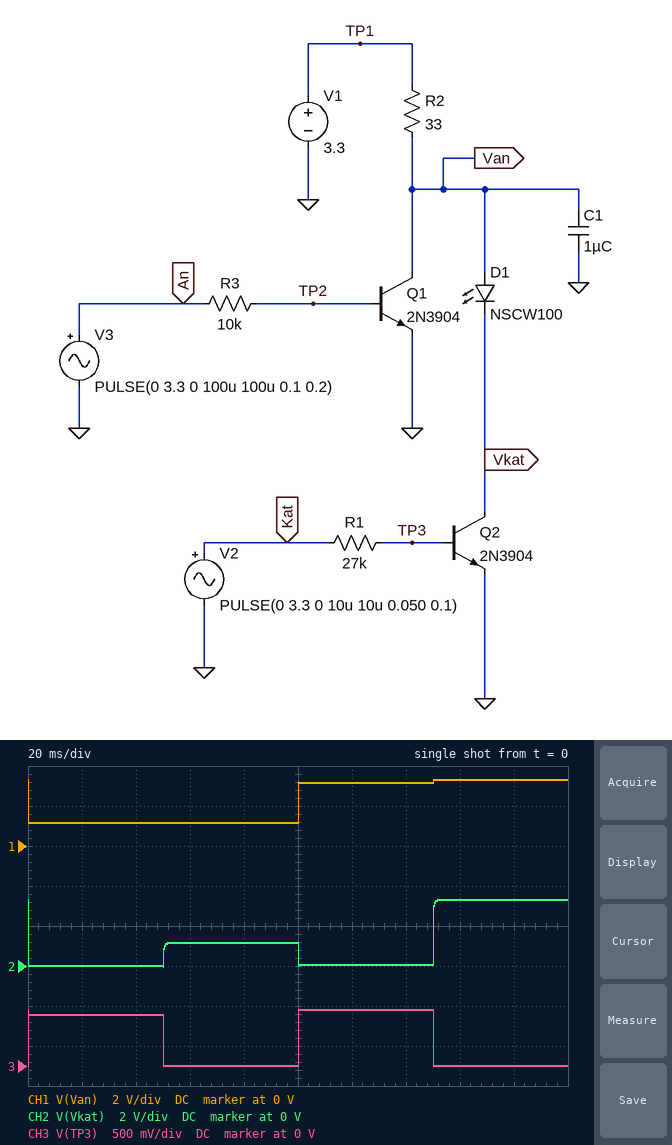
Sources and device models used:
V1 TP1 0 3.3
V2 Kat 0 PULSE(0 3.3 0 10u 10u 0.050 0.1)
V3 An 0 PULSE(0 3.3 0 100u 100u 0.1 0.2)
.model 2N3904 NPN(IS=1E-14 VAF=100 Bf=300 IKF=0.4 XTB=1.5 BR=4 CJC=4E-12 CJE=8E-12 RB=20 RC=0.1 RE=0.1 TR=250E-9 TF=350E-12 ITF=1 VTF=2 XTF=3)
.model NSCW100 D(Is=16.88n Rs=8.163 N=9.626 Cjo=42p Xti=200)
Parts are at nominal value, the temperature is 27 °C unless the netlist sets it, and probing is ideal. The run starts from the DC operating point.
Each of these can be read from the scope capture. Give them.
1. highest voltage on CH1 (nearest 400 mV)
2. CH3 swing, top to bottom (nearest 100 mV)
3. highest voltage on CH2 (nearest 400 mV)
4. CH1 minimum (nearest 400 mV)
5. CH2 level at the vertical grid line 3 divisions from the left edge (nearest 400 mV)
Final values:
3.2 V
700 mV
3.2 V
1.2 V
1.2 V
